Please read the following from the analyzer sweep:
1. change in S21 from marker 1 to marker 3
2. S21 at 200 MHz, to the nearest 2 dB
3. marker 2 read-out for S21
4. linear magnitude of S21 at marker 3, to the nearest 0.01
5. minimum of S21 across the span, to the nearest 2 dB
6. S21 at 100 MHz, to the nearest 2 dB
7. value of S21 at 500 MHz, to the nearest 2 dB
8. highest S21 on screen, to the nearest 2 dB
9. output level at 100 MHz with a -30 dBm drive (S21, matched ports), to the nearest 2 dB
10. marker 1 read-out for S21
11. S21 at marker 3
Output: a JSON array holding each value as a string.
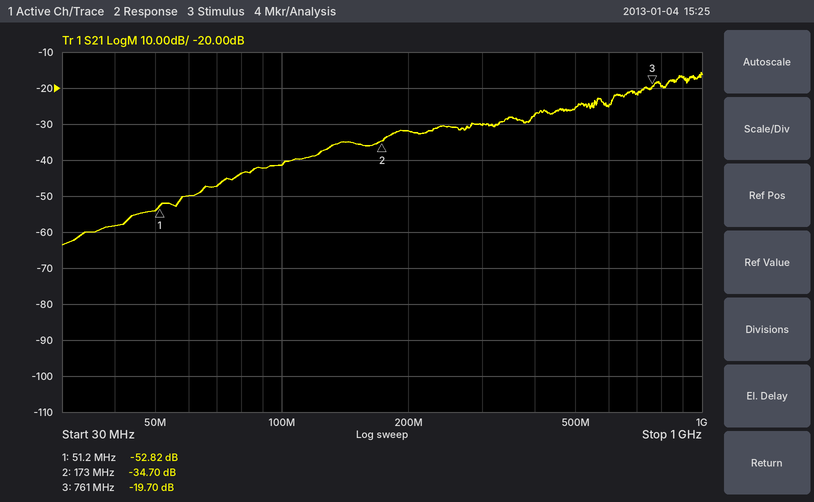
["33.12 dB", "-32 dB", "-34.70 dB", "0.10", "-64 dB", "-42 dB", "-26 dB", "-16 dB", "-72 dBm", "-52.82 dB", "-19.70 dB"]
